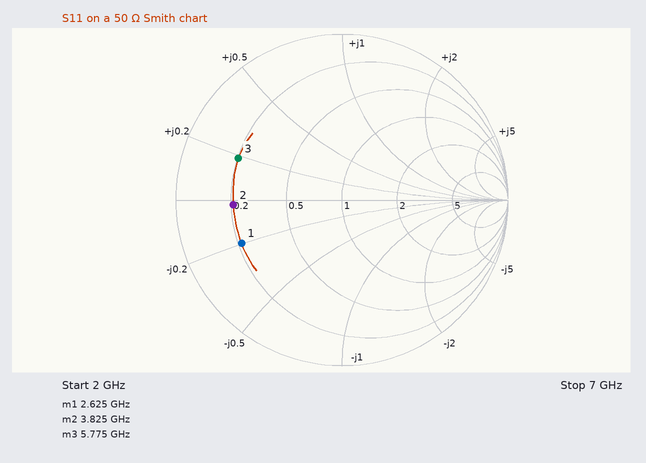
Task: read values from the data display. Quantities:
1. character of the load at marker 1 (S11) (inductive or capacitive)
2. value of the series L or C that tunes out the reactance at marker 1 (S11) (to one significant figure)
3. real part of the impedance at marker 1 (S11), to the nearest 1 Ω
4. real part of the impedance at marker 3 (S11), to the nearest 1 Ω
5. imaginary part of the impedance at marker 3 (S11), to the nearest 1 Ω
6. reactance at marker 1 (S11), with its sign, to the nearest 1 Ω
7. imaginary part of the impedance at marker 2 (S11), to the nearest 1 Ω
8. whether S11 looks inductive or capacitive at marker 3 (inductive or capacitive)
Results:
capacitive
600 pH
11 Ω
10 Ω
+9 Ω
-10 Ω
-1 Ω
inductive
